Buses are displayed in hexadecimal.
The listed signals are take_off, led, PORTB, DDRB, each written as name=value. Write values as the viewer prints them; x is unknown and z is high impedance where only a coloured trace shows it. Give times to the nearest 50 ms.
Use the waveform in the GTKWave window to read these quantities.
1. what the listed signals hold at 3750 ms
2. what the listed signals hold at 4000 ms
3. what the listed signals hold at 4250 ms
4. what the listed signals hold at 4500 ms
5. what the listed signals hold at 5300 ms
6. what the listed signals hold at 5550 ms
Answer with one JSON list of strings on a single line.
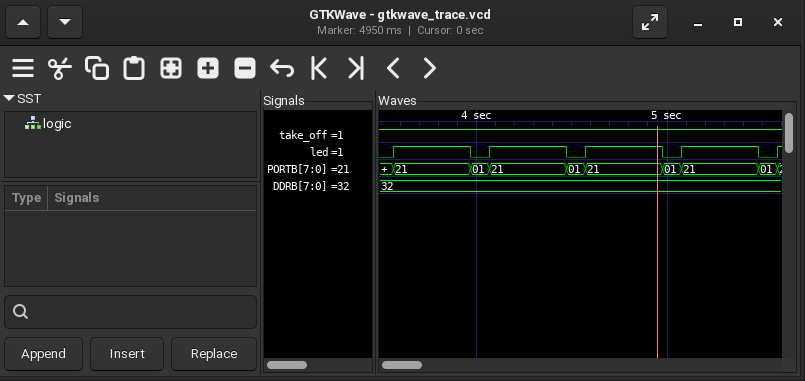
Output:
["take_off=1, led=1, PORTB=21, DDRB=32", "take_off=1, led=0, PORTB=01, DDRB=32", "take_off=1, led=1, PORTB=21, DDRB=32", "take_off=1, led=0, PORTB=01, DDRB=32", "take_off=1, led=1, PORTB=21, DDRB=32", "take_off=1, led=0, PORTB=01, DDRB=32"]
